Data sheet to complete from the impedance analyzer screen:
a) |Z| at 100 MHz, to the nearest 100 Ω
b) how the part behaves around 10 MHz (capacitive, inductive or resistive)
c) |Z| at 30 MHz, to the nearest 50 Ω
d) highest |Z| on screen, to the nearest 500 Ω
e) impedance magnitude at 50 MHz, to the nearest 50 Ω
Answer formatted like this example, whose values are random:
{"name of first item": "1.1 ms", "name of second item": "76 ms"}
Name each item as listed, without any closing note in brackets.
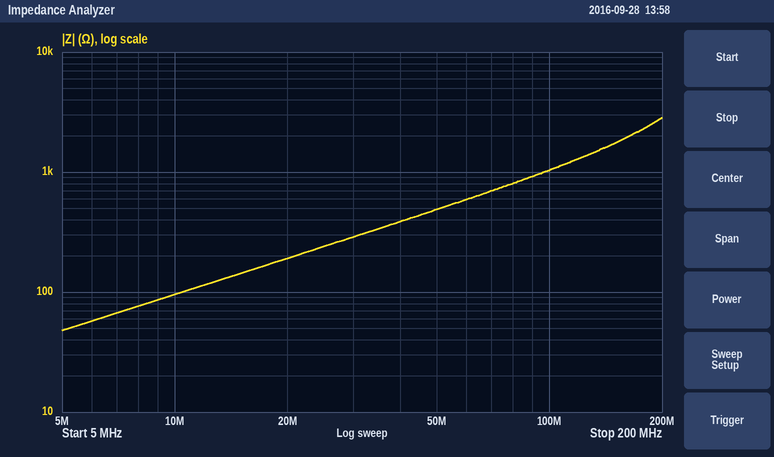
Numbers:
{"|Z| at 100 MHz, to the nearest 100 Ω": "1.0 kΩ", "how the part behaves around 10 MHz": "inductive", "|Z| at 30 MHz, to the nearest 50 Ω": "300 Ω", "highest |Z| on screen, to the nearest 500 Ω": "3.0 kΩ", "impedance magnitude at 50 MHz, to the nearest 50 Ω": "500 Ω"}
